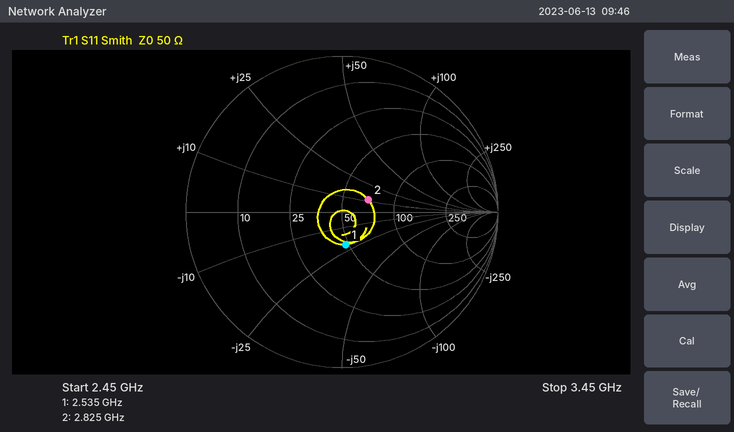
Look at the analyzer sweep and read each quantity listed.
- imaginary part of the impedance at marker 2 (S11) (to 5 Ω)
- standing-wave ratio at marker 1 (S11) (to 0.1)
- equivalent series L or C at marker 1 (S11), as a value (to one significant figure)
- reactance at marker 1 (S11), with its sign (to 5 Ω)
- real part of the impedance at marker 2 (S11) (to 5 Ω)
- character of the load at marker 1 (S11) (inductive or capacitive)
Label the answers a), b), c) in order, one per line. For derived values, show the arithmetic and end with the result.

a) +10 Ω
b) 1.5
c) C = 1/(2π × 2.535 GHz × 20 Ω) ≈ 3 pF
d) -20 Ω
e) 70 Ω
f) capacitive
